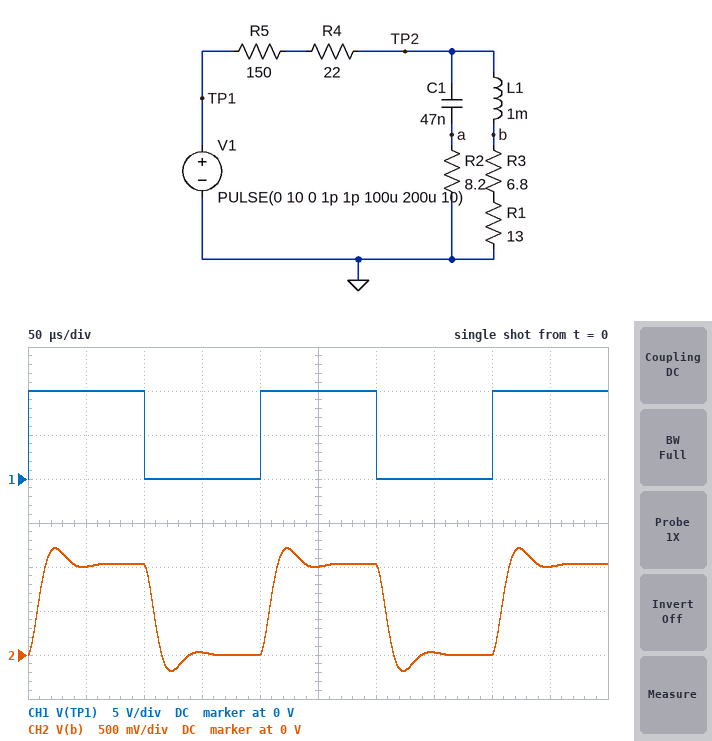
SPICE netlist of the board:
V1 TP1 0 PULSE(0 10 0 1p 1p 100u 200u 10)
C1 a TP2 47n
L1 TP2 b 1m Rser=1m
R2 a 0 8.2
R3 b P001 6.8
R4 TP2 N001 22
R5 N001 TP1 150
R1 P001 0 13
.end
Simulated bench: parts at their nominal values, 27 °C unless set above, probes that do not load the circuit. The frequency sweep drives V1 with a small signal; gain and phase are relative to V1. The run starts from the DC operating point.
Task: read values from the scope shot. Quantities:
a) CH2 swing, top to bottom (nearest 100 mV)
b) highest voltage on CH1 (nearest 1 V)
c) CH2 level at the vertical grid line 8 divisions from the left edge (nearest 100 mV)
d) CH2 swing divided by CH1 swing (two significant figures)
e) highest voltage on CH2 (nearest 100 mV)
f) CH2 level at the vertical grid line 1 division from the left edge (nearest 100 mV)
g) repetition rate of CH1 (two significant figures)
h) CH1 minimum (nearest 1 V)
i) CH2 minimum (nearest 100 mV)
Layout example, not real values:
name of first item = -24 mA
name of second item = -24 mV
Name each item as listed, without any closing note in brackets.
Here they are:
CH2 swing, top to bottom = 1.4 V
highest voltage on CH1 = 10 V
CH2 level at the vertical grid line 8 divisions from the left edge = 0 V
CH2 swing divided by CH1 swing = 0.14
highest voltage on CH2 = 1.2 V
CH2 level at the vertical grid line 1 division from the left edge = 1.0 V
repetition rate of CH1 = 5.0 kHz
CH1 minimum = 0 V
CH2 minimum = -200 mV
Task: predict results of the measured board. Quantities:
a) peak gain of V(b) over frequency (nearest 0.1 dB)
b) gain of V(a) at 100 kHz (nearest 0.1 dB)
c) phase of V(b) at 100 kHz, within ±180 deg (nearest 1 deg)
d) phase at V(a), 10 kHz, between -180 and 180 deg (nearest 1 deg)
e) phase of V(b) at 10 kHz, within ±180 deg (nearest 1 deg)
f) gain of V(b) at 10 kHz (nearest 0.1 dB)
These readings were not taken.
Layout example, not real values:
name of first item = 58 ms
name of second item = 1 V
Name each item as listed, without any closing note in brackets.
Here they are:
peak gain of V(b) over frequency = -18.3 dB
gain of V(a) at 100 kHz = -26.6 dB
phase of V(b) at 100 kHz, within ±180 deg = -153 deg
phase at V(a), 10 kHz, between -180 and 180 deg = 136 deg
phase of V(b) at 10 kHz, within ±180 deg = -25 deg
gain of V(b) at 10 kHz = -19.0 dB
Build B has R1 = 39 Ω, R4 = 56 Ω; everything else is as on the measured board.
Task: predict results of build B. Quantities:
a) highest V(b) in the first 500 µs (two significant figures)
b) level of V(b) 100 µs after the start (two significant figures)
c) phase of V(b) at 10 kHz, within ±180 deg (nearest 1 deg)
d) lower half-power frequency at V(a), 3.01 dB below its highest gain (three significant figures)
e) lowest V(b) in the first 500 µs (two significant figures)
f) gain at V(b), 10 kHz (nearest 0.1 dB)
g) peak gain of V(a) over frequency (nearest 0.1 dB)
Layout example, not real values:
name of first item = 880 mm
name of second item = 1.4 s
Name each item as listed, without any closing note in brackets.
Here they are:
highest V(b) in the first 500 µs = 2.1 V
level of V(b) 100 µs after the start = 1.8 V
phase of V(b) at 10 kHz, within ±180 deg = -23 deg
lower half-power frequency at V(a), 3.01 dB below its highest gain = 21.0 kHz
lowest V(b) in the first 500 µs = -320 mV
gain at V(b), 10 kHz = -14.1 dB
peak gain of V(a) over frequency = -26.7 dB
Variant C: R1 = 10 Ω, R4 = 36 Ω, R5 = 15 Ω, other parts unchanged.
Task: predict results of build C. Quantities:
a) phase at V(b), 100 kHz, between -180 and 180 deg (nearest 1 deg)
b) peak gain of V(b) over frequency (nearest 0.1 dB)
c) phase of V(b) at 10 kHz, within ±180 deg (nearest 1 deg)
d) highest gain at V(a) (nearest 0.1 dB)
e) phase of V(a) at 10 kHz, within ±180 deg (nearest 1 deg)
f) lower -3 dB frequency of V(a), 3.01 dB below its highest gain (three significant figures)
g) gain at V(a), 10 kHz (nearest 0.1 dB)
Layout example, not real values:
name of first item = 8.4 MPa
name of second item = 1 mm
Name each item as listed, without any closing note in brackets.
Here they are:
phase at V(b), 100 kHz, between -180 and 180 deg = -133 deg
peak gain of V(b) over frequency = -12.1 dB
phase of V(b) at 10 kHz, within ±180 deg = -48 deg
highest gain at V(a) = -17.2 dB
phase of V(a) at 10 kHz, within ±180 deg = 115 deg
lower -3 dB frequency of V(a), 3.01 dB below its highest gain = 51.2 kHz
gain at V(a), 10 kHz = -34.9 dB
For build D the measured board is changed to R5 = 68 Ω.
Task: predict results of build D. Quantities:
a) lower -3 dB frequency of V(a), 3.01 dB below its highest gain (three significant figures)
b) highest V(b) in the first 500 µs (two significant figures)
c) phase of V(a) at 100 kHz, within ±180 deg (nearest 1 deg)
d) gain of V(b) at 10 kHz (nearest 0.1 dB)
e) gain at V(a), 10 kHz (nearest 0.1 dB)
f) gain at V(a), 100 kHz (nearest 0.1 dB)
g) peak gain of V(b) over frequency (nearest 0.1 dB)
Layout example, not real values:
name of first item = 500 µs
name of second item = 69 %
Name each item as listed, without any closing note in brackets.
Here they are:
lower -3 dB frequency of V(a), 3.01 dB below its highest gain = 27.6 kHz
highest V(b) in the first 500 µs = 1.8 V
phase of V(a) at 100 kHz, within ±180 deg = 21 deg
gain of V(b) at 10 kHz = -15.3 dB
gain at V(a), 10 kHz = -37.2 dB
gain at V(a), 100 kHz = -21.7 dB
peak gain of V(b) over frequency = -14.9 dB
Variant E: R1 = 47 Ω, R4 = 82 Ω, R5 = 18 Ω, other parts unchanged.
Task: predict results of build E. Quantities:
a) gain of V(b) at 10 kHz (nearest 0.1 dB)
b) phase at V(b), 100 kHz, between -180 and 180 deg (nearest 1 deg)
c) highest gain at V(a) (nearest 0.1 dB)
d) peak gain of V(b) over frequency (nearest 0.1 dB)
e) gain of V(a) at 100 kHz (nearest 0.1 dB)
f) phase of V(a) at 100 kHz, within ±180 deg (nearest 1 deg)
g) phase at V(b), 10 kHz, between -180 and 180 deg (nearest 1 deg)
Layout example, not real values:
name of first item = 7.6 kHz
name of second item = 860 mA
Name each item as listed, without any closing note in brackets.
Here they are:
gain of V(b) at 10 kHz = -9.3 dB
phase at V(b), 100 kHz, between -180 and 180 deg = -142 deg
highest gain at V(a) = -22.4 dB
peak gain of V(b) over frequency = -9.1 dB
gain of V(a) at 100 kHz = -22.5 dB
phase of V(a) at 100 kHz, within ±180 deg = 19 deg
phase at V(b), 10 kHz, between -180 and 180 deg = -30 deg
